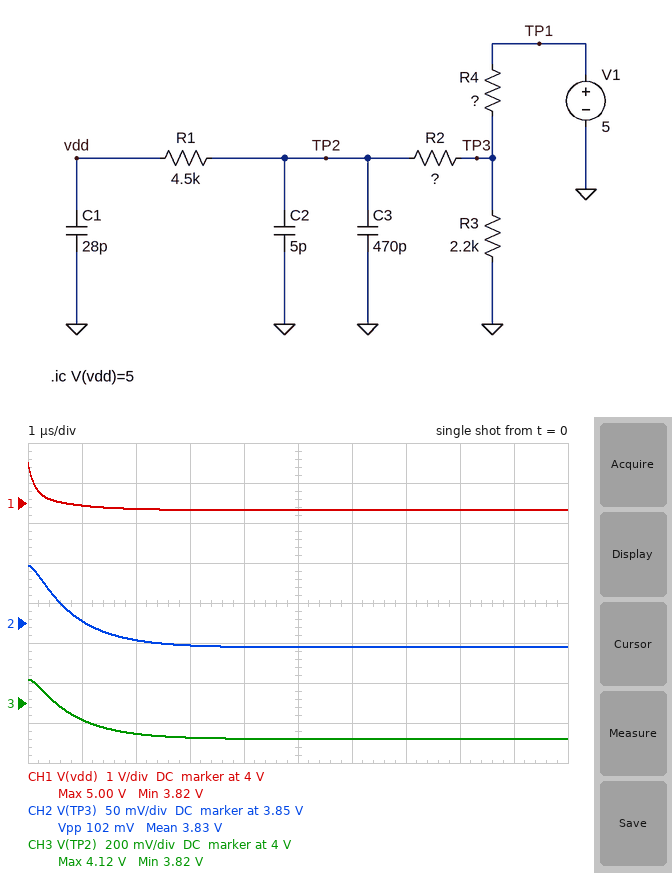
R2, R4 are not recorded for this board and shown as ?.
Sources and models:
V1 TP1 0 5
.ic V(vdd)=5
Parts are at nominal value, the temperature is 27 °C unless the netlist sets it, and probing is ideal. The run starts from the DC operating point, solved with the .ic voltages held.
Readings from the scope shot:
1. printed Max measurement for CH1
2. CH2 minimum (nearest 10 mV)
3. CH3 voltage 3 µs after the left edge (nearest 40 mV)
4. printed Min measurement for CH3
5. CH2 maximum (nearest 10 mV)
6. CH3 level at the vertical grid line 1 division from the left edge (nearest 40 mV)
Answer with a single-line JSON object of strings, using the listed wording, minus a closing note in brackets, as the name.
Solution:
{"printed Max measurement for CH1": "5.00 V", "CH2 minimum": "3.82 V", "CH3 voltage 3 µs after the left edge": "3.84 V", "printed Min measurement for CH3": "3.82 V", "CH2 maximum": "3.92 V", "CH3 level at the vertical grid line 1 division from the left edge": "3.92 V"}
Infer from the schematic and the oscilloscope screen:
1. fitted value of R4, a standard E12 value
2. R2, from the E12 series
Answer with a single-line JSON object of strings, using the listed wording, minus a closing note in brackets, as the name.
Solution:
{"fitted value of R4, a standard E12 value": "680 Ω", "R2, from the E12 series": "1 kΩ"}
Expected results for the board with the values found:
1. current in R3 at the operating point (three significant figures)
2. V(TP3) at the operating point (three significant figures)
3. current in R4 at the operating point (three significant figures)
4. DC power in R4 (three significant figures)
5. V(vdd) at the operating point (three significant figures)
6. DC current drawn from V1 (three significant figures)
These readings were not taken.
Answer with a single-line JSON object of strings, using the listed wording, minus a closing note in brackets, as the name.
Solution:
{"current in R3 at the operating point": "1.74 mA", "V(TP3) at the operating point": "3.82 V", "current in R4 at the operating point": "1.74 mA", "DC power in R4": "2.05 mW", "V(vdd) at the operating point": "3.82 V", "DC current drawn from V1": "1.74 mA"}
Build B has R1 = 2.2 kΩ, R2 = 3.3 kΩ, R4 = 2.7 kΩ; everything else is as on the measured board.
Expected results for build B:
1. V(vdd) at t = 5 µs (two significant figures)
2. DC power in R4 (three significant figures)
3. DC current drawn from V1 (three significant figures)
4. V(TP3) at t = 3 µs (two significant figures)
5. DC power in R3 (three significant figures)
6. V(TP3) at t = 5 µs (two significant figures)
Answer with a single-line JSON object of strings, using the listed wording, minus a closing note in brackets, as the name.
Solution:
{"V(vdd) at t = 5 µs": "2.5 V", "DC power in R4": "2.81 mW", "DC current drawn from V1": "1.02 mA", "V(TP3) at t = 3 µs": "2.4 V", "DC power in R3": "2.29 mW", "V(TP3) at t = 5 µs": "2.3 V"}
